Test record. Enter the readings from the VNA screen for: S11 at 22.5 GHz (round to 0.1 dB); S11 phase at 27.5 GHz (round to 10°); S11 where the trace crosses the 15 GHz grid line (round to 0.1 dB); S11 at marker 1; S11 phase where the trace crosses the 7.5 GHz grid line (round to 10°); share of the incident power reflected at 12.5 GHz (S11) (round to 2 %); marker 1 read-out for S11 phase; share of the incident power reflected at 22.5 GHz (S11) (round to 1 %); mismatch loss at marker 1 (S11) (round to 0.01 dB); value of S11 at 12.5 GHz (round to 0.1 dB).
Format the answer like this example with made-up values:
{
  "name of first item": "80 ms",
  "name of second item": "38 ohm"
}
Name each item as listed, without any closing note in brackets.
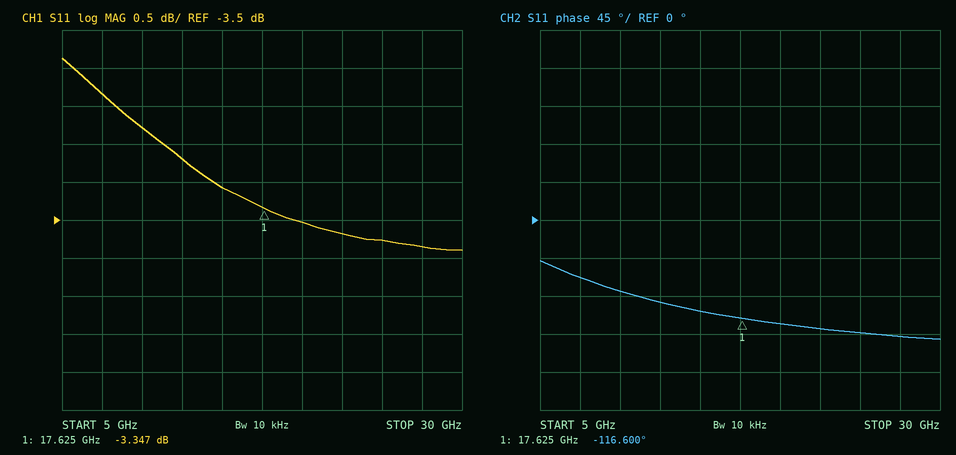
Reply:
{
  "S11 at 22.5 GHz": "-3.7 dB",
  "S11 phase at 27.5 GHz": "-140°",
  "S11 where the trace crosses the 15 GHz grid line": "-3.1 dB",
  "S11 at marker 1": "-3.347 dB",
  "S11 phase where the trace crosses the 7.5 GHz grid line": "-70°",
  "share of the incident power reflected at 12.5 GHz (S11)": "54 %",
  "marker 1 read-out for S11 phase": "-116.600°",
  "share of the incident power reflected at 22.5 GHz (S11)": "43 %",
  "mismatch loss at marker 1 (S11)": "2.70 dB",
  "value of S11 at 12.5 GHz": "-2.7 dB"
}
